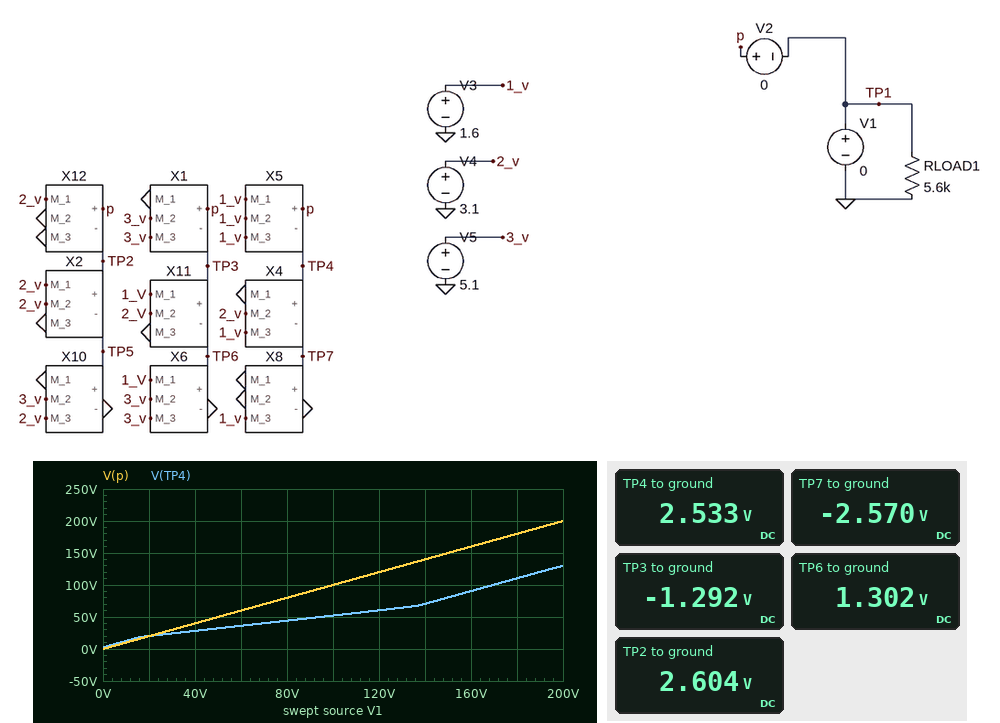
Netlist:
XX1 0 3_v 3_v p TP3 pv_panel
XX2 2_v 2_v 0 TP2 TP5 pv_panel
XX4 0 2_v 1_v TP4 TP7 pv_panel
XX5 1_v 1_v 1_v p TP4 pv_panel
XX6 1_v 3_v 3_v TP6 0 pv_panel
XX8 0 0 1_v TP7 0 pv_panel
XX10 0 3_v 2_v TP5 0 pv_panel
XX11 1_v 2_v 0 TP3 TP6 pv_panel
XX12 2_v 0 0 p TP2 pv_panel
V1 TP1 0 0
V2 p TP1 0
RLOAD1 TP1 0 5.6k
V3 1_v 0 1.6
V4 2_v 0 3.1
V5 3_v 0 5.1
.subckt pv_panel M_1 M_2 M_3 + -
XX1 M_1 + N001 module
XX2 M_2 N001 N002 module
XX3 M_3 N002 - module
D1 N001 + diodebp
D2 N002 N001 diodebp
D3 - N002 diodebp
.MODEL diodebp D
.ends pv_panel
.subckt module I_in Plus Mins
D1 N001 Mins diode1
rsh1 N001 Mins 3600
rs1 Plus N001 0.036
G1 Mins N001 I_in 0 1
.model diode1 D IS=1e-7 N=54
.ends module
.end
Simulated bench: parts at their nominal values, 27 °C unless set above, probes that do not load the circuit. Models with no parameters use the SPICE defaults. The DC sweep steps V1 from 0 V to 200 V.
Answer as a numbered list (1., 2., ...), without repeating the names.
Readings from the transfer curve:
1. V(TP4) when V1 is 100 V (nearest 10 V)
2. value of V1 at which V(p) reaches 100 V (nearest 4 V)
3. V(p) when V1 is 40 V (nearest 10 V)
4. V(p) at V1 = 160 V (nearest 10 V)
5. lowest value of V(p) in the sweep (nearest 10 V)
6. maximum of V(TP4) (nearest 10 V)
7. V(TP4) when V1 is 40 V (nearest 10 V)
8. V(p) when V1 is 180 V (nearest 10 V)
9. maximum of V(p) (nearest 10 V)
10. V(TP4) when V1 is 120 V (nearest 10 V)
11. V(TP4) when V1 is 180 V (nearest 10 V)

1. 50 V
2. 100 V
3. 40 V
4. 160 V
5. 0 V
6. 130 V
7. 30 V
8. 180 V
9. 200 V
10. 60 V
11. 110 V
